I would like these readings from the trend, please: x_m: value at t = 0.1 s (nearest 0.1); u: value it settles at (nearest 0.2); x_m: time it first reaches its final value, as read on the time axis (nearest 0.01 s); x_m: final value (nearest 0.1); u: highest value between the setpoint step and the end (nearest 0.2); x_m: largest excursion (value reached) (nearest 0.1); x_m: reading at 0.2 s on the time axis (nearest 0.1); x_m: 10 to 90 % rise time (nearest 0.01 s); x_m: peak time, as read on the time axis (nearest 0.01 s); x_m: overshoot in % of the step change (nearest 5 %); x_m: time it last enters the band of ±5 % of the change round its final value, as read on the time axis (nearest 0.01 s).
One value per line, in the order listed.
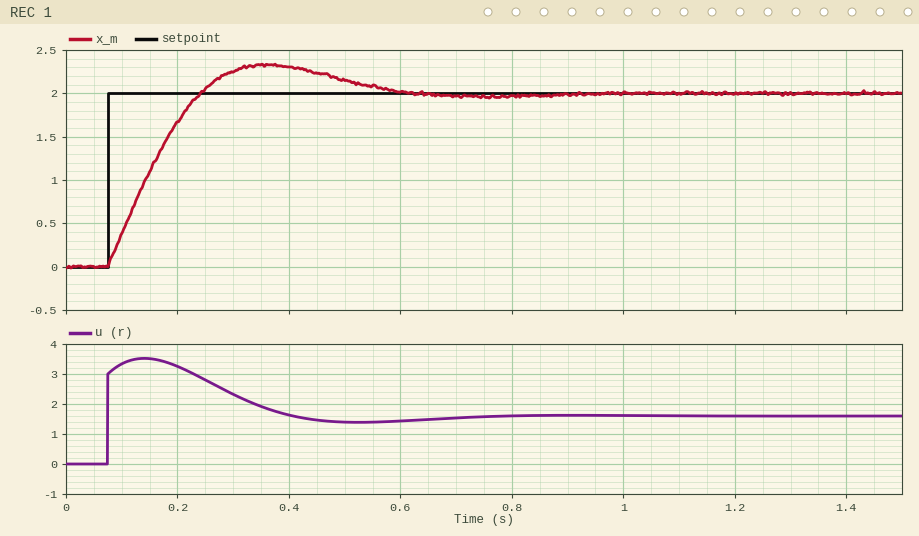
0.4
1.6
0.24 s
2.0
3.6
2.3
1.7
0.13 s
0.36 s
15 %
0.53 s
